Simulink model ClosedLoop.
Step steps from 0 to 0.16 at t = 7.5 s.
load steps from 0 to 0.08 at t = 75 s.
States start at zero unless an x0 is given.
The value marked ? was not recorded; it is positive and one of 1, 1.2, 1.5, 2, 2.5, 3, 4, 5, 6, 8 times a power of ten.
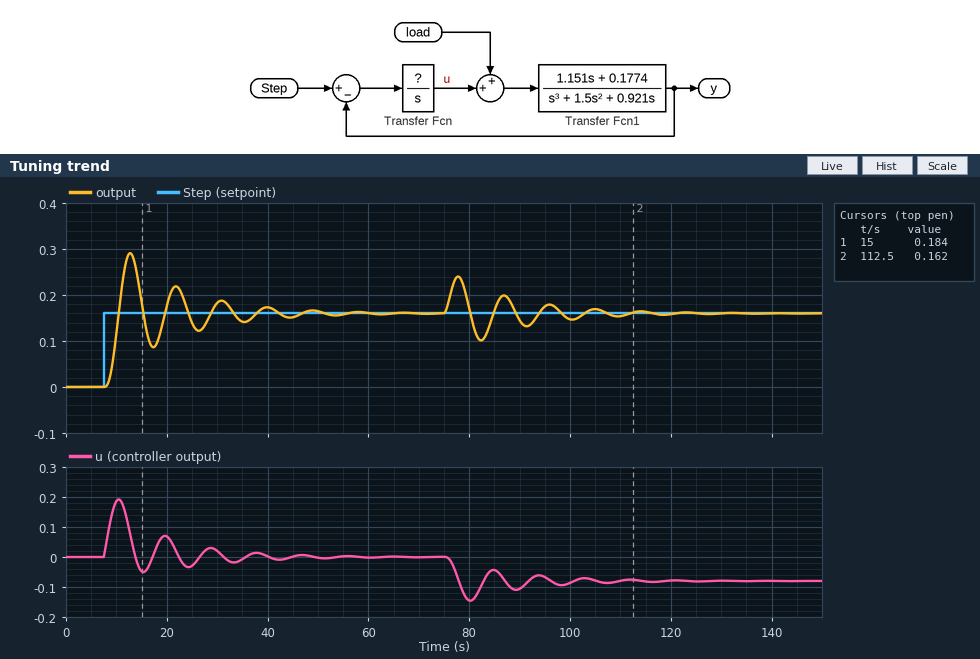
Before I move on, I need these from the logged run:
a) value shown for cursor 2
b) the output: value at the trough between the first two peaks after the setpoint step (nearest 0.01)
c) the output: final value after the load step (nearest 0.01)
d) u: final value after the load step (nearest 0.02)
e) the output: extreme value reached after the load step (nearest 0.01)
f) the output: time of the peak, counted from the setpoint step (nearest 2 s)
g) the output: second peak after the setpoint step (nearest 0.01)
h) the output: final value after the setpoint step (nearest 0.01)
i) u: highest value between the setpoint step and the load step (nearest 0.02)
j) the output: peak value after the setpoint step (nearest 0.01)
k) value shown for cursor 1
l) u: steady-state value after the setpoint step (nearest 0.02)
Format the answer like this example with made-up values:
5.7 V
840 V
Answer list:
0.162
0.09
0.16
-0.08
0.24
6 s
0.22
0.16
0.20
0.29
0.184
0.00
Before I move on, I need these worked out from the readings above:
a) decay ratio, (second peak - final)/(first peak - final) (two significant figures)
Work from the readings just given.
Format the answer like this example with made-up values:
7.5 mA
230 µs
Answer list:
0.46
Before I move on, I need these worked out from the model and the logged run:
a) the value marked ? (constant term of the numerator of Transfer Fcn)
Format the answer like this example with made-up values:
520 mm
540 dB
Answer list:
0.6
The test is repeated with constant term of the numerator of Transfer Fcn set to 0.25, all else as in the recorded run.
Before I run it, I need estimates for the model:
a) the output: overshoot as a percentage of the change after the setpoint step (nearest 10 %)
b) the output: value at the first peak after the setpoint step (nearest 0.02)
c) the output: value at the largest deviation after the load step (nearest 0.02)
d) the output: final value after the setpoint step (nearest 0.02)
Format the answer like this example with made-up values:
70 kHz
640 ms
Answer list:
50 %
0.24
0.26
0.16
